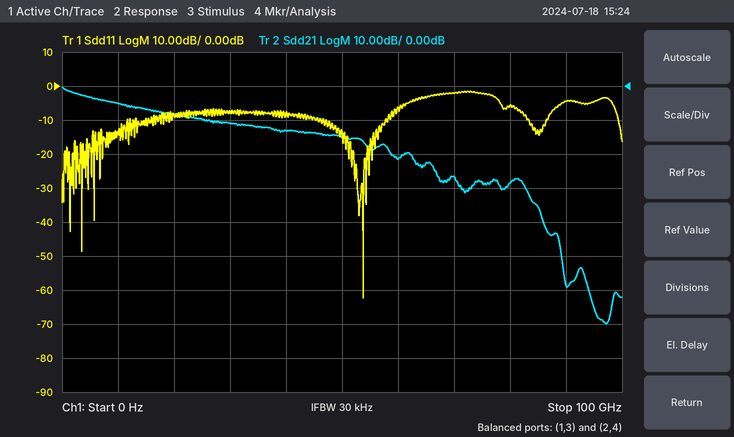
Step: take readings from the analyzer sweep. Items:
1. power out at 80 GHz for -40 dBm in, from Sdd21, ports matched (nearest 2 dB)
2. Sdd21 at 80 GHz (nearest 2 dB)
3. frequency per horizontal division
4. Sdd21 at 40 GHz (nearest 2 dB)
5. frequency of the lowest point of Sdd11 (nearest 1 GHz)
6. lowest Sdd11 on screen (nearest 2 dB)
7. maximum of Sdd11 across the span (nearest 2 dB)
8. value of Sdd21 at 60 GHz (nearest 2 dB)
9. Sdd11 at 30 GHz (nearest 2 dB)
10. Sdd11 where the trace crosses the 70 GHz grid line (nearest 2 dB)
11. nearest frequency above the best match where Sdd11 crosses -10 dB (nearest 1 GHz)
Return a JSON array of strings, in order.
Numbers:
["-68 dBm", "-28 dB", "10 GHz", "-14 dB", "54 GHz", "-62 dB", "-2 dB", "-22 dB", "-8 dB", "-2 dB", "58 GHz"]
